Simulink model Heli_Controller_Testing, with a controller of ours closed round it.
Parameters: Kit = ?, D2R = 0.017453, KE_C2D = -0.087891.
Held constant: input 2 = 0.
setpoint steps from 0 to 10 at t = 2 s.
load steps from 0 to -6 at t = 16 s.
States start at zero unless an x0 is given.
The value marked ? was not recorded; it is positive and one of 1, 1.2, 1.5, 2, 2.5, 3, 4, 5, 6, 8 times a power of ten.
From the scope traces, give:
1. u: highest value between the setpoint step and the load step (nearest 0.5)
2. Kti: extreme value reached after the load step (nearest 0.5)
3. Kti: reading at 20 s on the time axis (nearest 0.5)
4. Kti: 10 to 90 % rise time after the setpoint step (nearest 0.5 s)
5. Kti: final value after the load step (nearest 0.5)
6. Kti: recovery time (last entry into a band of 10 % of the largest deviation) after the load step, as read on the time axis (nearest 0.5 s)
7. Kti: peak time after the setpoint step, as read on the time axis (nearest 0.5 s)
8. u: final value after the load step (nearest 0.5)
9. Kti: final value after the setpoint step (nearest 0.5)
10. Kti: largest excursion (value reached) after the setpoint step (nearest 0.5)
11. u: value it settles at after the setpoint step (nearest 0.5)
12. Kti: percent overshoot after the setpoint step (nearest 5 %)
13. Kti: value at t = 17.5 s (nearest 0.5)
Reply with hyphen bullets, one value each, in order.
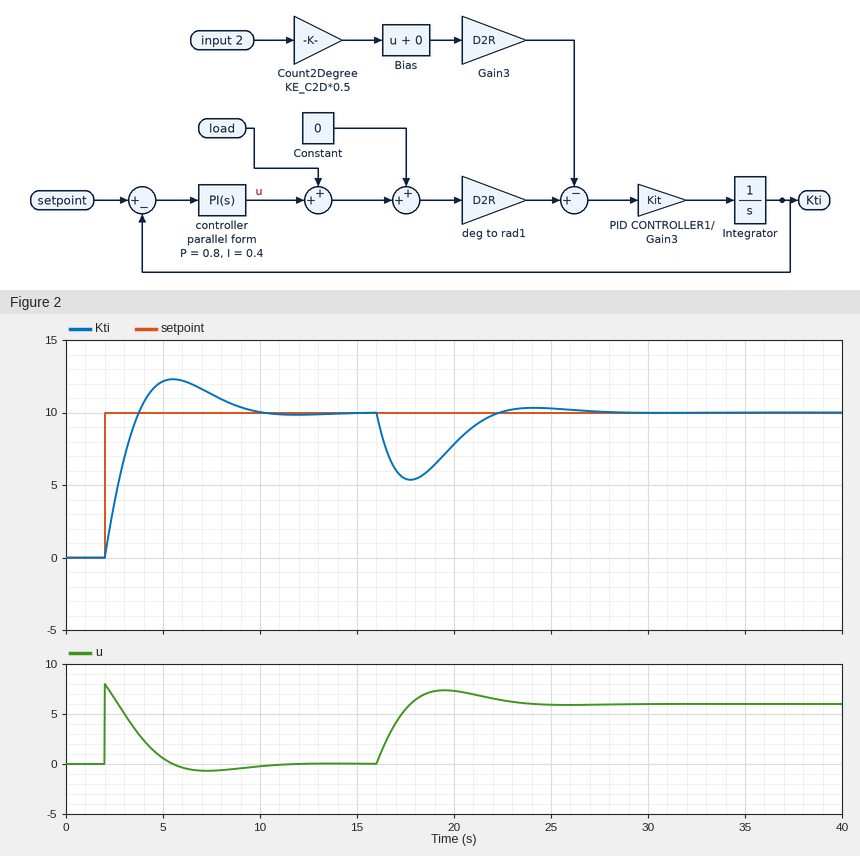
- 8.0
- 5.5
- 8.0
- 1.5 s
- 10.0
- 21.5 s
- 5.5 s
- 6.0
- 10.0
- 12.5
- 0.0
- 25 %
- 5.5
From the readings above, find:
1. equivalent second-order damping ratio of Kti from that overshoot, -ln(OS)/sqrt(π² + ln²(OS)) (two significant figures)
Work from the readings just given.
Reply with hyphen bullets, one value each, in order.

- 0.40
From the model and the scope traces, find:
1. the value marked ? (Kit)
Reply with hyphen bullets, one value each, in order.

- 60
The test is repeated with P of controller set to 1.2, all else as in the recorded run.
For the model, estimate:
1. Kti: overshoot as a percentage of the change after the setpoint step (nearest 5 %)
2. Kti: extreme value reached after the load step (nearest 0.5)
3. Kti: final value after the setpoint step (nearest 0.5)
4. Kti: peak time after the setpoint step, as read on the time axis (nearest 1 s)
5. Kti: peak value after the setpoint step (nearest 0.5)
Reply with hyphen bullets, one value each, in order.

- 15 %
- 6.5
- 10.0
- 5 s
- 11.5
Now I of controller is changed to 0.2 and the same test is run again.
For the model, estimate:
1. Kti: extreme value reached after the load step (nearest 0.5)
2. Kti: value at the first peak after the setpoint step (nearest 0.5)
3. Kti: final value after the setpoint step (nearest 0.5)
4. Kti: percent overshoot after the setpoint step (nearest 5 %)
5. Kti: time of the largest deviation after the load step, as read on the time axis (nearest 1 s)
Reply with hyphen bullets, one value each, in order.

- 4.5
- 11.5
- 10.0
- 15 %
- 18 s
